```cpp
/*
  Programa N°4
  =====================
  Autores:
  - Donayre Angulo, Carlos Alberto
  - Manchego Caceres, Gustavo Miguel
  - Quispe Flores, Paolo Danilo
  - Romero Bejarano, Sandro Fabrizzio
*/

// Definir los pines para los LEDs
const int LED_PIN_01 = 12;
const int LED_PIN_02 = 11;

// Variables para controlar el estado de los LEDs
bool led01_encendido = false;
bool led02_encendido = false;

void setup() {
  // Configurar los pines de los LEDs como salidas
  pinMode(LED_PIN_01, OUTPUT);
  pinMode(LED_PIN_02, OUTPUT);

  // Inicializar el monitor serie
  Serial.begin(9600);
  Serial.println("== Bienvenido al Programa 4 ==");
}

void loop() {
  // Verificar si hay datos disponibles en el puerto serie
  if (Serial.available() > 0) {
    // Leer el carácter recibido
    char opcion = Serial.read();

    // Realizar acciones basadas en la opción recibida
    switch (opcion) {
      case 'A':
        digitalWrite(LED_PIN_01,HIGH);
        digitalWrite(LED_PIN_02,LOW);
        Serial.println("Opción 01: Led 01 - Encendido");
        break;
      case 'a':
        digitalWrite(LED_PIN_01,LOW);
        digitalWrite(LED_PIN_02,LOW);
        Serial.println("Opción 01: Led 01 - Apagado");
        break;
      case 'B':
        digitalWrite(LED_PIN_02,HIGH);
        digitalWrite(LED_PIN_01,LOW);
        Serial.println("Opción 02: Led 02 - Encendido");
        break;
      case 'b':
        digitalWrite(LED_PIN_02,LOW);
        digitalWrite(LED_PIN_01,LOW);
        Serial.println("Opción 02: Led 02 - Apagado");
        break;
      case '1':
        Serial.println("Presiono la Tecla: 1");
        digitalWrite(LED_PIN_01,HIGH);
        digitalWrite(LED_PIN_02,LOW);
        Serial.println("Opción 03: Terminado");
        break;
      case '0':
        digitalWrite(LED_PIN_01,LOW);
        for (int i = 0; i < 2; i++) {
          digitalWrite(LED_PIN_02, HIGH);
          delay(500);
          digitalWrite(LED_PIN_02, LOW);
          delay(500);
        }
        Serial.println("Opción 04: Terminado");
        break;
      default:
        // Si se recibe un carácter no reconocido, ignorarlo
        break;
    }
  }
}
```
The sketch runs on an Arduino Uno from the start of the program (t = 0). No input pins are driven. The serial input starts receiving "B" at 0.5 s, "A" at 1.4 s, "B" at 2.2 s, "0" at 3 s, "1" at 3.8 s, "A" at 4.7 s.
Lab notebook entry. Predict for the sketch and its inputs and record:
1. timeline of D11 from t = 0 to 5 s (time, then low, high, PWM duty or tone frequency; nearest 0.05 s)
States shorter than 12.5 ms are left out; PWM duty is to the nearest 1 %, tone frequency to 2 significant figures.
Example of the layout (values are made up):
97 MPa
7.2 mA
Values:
0 s low; 0.5 s high; 1.4 s low; 2.2 s high; 3.5 s low; 4 s high; 4.5 s low
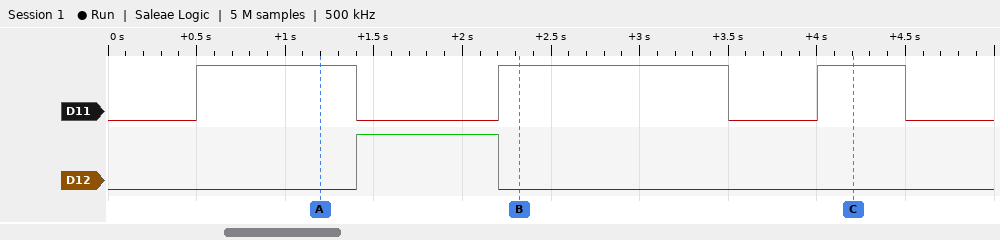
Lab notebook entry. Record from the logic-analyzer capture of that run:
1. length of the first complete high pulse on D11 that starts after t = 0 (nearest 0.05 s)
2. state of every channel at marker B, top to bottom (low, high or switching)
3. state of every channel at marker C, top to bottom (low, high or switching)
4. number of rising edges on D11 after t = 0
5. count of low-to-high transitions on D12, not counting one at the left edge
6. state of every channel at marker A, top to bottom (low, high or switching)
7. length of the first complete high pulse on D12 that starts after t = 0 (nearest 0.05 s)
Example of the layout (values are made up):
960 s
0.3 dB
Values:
0.90 s
D11 high, D12 low
D11 high, D12 low
3
1
D11 high, D12 low
0.80 s
